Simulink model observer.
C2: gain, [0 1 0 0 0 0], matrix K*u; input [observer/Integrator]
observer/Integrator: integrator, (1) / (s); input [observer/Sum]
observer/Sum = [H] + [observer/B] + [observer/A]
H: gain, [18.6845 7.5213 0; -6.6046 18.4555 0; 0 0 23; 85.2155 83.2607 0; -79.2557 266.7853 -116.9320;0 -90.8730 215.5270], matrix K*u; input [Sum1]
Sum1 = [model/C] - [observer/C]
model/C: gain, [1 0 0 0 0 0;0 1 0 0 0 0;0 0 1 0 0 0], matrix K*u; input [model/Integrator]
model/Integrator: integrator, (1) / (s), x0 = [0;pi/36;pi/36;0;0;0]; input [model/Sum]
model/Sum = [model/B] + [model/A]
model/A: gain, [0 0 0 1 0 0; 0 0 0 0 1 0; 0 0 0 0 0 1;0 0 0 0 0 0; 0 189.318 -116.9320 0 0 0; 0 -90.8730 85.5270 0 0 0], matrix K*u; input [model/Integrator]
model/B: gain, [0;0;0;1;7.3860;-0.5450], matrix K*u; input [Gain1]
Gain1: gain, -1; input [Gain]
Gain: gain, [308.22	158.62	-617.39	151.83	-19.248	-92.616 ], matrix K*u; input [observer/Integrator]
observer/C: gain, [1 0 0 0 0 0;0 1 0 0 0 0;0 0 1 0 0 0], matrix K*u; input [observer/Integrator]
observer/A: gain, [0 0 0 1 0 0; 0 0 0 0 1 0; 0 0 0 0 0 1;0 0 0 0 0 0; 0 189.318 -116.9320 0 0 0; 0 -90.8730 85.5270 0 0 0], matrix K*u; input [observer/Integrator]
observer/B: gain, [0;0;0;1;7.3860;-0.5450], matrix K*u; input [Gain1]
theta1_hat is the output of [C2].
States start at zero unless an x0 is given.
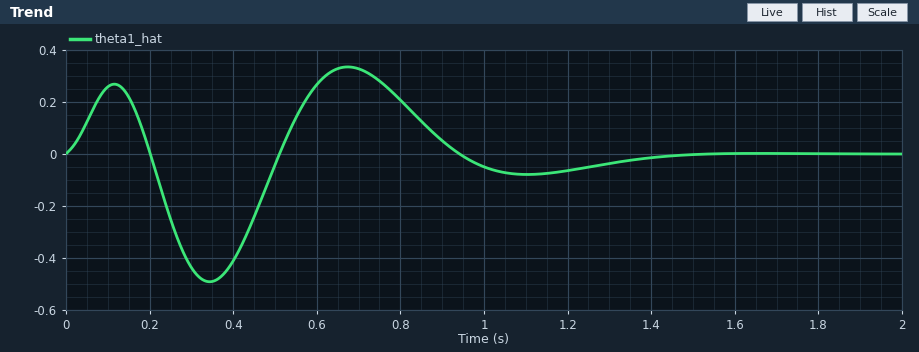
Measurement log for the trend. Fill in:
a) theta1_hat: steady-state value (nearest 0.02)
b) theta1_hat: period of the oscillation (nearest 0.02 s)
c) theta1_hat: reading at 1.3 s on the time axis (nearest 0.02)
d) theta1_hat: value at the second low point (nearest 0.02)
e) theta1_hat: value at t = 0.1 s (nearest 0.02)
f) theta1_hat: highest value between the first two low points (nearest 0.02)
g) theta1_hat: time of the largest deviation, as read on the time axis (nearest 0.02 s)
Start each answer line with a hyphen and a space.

- 0.00
- 0.76 s
- -0.04
- -0.08
- 0.26
- 0.34
- 0.34 s
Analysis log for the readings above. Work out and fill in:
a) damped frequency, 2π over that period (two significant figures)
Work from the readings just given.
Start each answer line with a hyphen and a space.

- 8.3 rad/s
